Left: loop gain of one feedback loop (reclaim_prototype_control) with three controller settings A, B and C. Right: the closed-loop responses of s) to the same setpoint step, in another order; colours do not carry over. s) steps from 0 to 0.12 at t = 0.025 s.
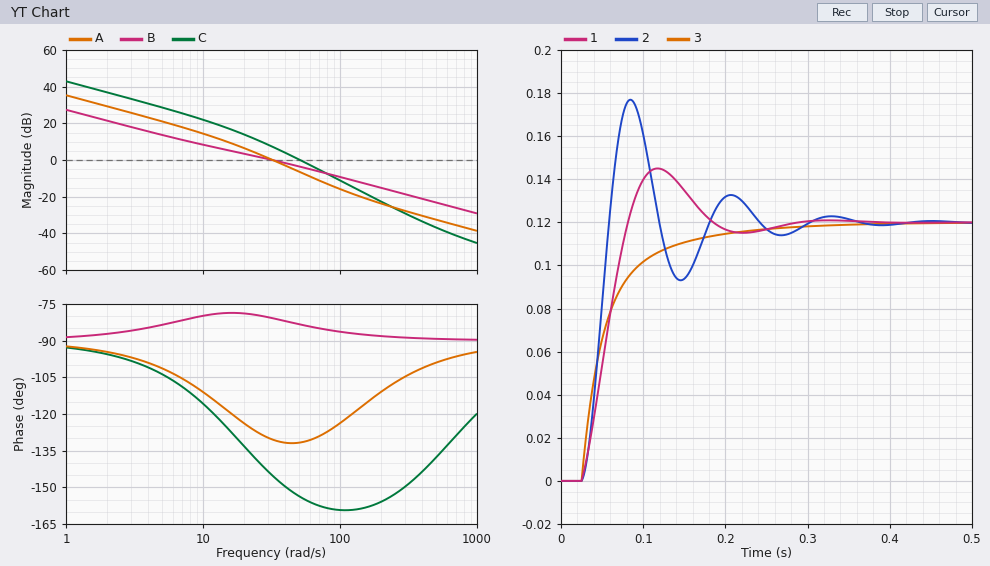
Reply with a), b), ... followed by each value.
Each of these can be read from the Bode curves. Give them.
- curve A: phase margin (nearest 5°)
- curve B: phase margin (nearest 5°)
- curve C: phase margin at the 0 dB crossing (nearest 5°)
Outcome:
a) 50°
b) 100°
c) 25°
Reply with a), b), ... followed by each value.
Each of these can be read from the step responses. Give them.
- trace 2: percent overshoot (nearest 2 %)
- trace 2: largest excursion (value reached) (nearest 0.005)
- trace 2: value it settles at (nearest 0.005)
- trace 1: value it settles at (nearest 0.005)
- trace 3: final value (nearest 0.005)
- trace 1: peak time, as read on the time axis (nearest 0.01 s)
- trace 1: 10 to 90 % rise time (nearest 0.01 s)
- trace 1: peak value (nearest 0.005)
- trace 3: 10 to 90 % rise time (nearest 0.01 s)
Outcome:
a) 48 %
b) 0.175
c) 0.120
d) 0.120
e) 0.120
f) 0.12 s
g) 0.04 s
h) 0.145
i) 0.10 s
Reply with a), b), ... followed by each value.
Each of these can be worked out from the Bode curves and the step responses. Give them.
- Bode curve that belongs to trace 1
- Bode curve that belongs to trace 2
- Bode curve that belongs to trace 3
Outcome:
a) A
b) C
c) B
